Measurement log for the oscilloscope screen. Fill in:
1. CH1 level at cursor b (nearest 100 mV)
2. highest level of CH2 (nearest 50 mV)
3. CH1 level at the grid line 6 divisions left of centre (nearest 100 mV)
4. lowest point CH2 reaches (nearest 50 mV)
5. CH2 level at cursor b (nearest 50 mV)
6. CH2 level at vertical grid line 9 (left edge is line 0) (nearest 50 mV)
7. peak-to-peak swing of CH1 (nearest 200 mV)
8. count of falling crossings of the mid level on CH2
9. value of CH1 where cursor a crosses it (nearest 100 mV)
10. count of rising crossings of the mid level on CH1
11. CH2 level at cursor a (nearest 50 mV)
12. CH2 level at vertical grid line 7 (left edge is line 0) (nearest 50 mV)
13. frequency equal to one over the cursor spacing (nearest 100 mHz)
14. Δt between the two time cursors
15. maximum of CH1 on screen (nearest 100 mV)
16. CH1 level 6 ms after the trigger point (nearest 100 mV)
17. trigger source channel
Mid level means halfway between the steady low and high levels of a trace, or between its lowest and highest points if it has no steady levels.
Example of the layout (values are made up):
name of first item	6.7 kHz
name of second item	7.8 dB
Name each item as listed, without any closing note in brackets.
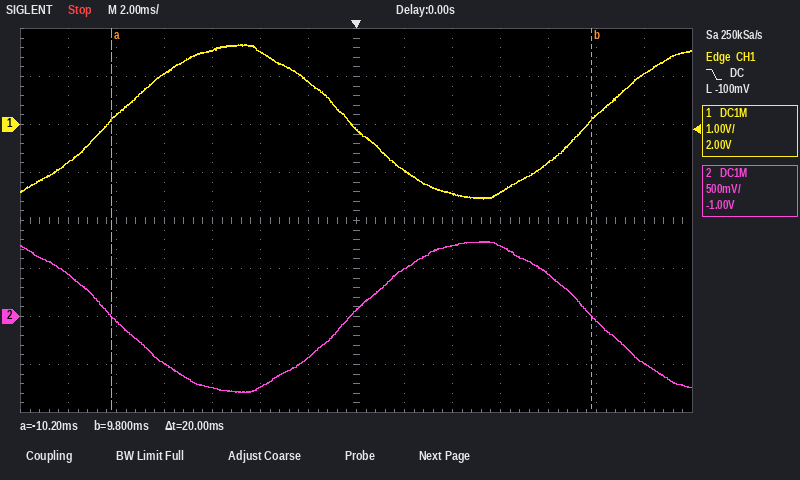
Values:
CH1 level at cursor b	100 mV
highest level of CH2	800 mV
CH1 level at the grid line 6 divisions left of centre	-800 mV
lowest point CH2 reaches	-800 mV
CH2 level at cursor b	0 mV
CH2 level at vertical grid line 9 (left edge is line 0)	750 mV
peak-to-peak swing of CH1	3.2 V
count of falling crossings of the mid level on CH2	2
value of CH1 where cursor a crosses it	100 mV
count of rising crossings of the mid level on CH1	2
CH2 level at cursor a	0 mV
CH2 level at vertical grid line 7 (left edge is line 0)	50 mV
frequency equal to one over the cursor spacing	50.0 Hz
Δt between the two time cursors	20 ms
maximum of CH1 on screen	1.7 V
CH1 level 6 ms after the trigger point	-1.4 V
trigger source channel	CH1
